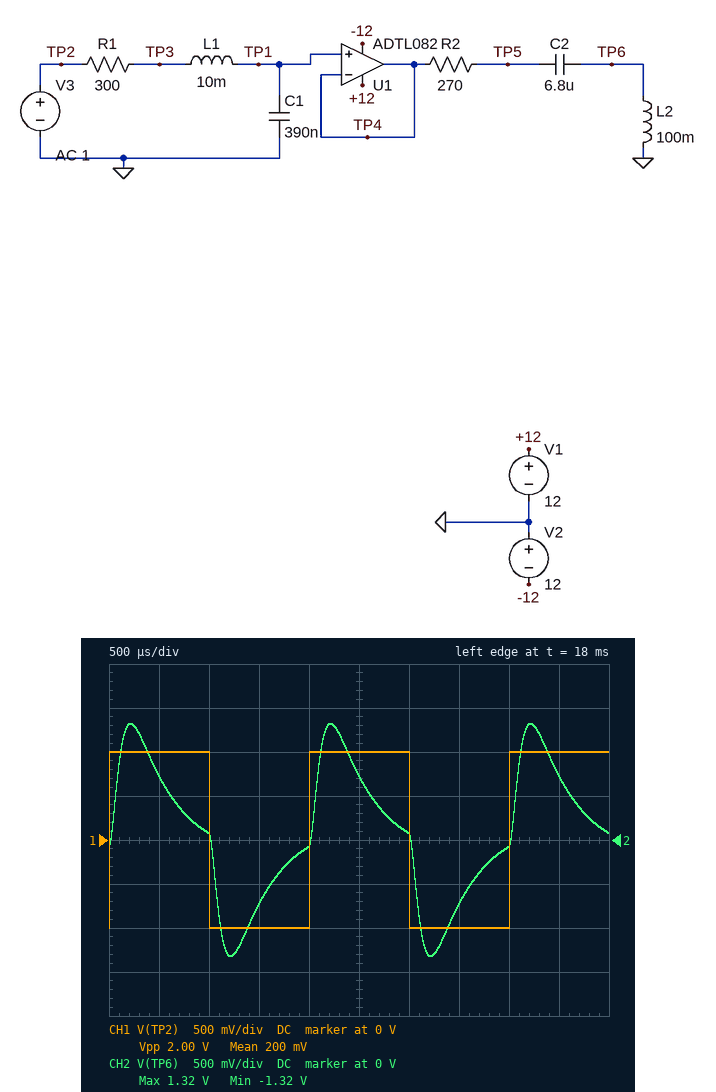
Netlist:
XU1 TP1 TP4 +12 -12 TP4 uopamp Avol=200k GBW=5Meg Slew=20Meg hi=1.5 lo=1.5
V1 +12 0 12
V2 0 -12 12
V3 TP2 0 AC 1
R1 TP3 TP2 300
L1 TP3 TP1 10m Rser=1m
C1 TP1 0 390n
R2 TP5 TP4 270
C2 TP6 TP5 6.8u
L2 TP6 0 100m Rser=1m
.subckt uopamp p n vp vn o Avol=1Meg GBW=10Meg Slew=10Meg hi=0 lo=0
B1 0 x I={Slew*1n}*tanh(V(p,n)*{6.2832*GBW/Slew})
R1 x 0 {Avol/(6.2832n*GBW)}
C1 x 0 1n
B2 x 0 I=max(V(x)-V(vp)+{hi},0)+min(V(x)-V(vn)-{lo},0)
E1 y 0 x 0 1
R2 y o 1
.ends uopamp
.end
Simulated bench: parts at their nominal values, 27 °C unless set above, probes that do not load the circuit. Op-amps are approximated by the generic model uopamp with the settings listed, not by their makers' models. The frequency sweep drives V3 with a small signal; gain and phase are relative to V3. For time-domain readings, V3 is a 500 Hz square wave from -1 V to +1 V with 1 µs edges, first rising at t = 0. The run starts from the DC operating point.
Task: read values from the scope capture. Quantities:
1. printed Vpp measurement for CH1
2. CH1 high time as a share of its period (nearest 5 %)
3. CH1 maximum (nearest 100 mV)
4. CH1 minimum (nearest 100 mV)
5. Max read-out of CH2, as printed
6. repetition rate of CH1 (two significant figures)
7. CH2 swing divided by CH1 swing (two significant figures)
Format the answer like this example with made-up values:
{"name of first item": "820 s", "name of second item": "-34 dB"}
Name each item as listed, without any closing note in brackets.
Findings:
{"printed Vpp measurement for CH1": "2.00 V", "CH1 high time as a share of its period": "50 %", "CH1 maximum": "1.0 V", "CH1 minimum": "-1.0 V", "Max read-out of CH2, as printed": "1.32 V", "repetition rate of CH1": "500 Hz", "CH2 swing divided by CH1 swing": "1.3"}
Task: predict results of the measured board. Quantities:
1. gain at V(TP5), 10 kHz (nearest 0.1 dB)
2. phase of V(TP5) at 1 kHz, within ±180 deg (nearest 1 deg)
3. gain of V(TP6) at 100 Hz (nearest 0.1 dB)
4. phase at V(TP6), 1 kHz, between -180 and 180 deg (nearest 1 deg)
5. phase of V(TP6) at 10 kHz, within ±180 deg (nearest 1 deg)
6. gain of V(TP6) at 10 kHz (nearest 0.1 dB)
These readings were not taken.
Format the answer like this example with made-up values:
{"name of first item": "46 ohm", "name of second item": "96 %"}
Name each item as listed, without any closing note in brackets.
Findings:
{"gain at V(TP5), 10 kHz": "-24.2 dB", "phase of V(TP5) at 1 kHz, within ±180 deg": "-17 deg", "gain of V(TP6) at 100 Hz": "-14.1 dB", "phase at V(TP6), 1 kHz, between -180 and 180 deg": "-17 deg", "phase of V(TP6) at 10 kHz, within ±180 deg": "-151 deg", "gain of V(TP6) at 10 kHz": "-24.2 dB"}
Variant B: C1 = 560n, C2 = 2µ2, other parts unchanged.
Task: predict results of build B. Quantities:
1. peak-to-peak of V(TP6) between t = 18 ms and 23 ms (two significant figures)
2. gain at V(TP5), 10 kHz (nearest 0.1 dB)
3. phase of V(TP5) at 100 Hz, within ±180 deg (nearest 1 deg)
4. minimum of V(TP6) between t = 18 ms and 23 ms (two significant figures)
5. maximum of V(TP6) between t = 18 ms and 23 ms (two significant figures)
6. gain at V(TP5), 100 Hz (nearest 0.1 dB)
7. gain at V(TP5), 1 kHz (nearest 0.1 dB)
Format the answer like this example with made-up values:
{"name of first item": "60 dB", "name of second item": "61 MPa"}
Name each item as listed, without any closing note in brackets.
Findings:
{"peak-to-peak of V(TP6) between t = 18 ms and 23 ms": "2.8 V", "gain at V(TP5), 10 kHz": "-27.5 dB", "phase of V(TP5) at 100 Hz, within ±180 deg": "-28 deg", "minimum of V(TP6) between t = 18 ms and 23 ms": "-1.4 V", "maximum of V(TP6) between t = 18 ms and 23 ms": "1.4 V", "gain at V(TP5), 100 Hz": "-0.7 dB", "gain at V(TP5), 1 kHz": "-3.3 dB"}
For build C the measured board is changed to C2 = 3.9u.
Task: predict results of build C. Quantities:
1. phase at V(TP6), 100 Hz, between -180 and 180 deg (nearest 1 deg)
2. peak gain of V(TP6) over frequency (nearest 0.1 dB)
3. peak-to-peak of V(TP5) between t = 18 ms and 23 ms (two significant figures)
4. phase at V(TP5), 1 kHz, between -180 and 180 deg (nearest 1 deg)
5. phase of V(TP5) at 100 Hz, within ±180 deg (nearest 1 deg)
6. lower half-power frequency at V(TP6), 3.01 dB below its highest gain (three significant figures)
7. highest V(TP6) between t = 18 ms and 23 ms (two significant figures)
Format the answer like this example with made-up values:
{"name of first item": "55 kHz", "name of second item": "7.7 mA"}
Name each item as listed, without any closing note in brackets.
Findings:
{"phase at V(TP6), 100 Hz, between -180 and 180 deg": "138 deg", "peak gain of V(TP6) over frequency": "-1.0 dB", "peak-to-peak of V(TP5) between t = 18 ms and 23 ms": "2.3 V", "phase at V(TP5), 1 kHz, between -180 and 180 deg": "-16 deg", "phase of V(TP5) at 100 Hz, within ±180 deg": "-42 deg", "lower half-power frequency at V(TP6), 3.01 dB below its highest gain": "274 Hz", "highest V(TP6) between t = 18 ms and 23 ms": "1.4 V"}
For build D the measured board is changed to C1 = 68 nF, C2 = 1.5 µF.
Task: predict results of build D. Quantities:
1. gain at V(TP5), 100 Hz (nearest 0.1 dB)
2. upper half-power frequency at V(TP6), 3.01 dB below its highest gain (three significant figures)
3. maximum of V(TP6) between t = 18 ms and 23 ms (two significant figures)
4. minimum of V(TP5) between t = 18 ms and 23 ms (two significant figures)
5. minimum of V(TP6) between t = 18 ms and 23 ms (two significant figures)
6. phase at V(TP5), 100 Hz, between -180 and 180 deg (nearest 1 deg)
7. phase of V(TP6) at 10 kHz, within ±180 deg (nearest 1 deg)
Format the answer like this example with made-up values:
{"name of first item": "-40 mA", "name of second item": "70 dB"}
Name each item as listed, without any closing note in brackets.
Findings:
{"gain at V(TP5), 100 Hz": "-0.3 dB", "upper half-power frequency at V(TP6), 3.01 dB below its highest gain": "7.25 kHz", "maximum of V(TP6) between t = 18 ms and 23 ms": "2.8 V", "minimum of V(TP5) between t = 18 ms and 23 ms": "-1.8 V", "minimum of V(TP6) between t = 18 ms and 23 ms": "-2.8 V", "phase at V(TP5), 100 Hz, between -180 and 180 deg": "-16 deg", "phase of V(TP6) at 10 kHz, within ±180 deg": "-140 deg"}
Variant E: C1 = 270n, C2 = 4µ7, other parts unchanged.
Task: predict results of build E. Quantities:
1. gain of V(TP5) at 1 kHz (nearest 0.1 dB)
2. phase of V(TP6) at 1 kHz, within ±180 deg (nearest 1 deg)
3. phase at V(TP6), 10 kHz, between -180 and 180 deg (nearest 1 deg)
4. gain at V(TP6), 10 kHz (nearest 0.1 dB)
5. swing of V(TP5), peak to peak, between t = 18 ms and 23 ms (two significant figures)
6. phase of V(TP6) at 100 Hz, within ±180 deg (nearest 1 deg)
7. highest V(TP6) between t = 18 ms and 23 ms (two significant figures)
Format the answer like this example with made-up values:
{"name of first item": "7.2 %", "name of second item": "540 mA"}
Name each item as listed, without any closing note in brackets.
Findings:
{"gain of V(TP5) at 1 kHz": "-1.1 dB", "phase of V(TP6) at 1 kHz, within ±180 deg": "-5 deg", "phase at V(TP6), 10 kHz, between -180 and 180 deg": "-150 deg", "gain at V(TP6), 10 kHz": "-20.8 dB", "swing of V(TP5), peak to peak, between t = 18 ms and 23 ms": "2.7 V", "phase of V(TP6) at 100 Hz, within ±180 deg": "133 deg", "highest V(TP6) between t = 18 ms and 23 ms": "1.6 V"}
